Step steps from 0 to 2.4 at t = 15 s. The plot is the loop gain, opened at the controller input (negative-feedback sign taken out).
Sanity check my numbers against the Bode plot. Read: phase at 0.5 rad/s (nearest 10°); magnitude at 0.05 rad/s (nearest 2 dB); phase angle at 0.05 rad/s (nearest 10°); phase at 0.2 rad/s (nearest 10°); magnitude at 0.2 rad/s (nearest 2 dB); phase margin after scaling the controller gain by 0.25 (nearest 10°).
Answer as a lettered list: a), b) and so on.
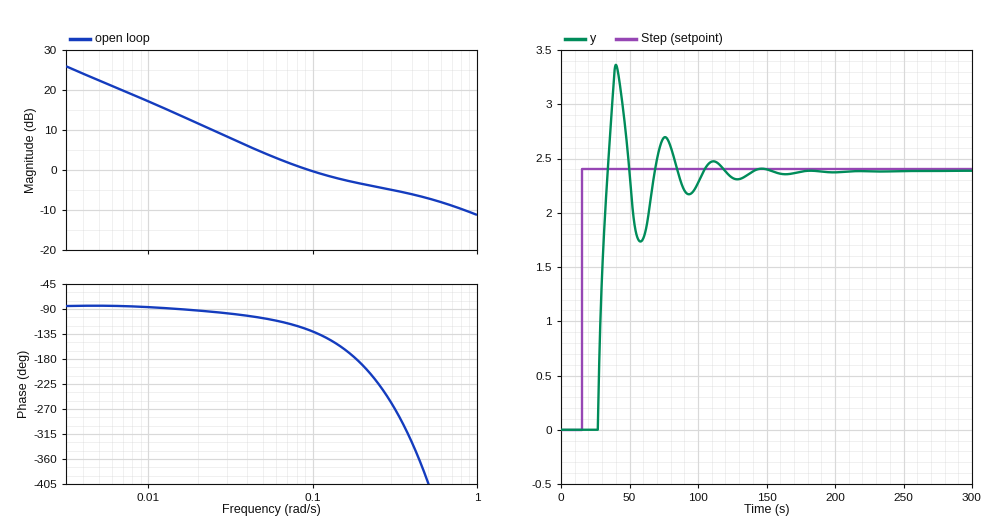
a) -400°
b) 4 dB
c) -110°
d) -190°
e) -4 dB
f) 90°
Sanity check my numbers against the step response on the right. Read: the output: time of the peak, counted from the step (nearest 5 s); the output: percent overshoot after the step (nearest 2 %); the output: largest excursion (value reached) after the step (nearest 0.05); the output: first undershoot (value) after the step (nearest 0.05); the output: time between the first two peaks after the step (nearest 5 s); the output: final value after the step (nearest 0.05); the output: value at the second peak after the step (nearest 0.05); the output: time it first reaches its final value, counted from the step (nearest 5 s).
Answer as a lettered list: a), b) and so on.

a) 25 s
b) 40 %
c) 3.35
d) 1.75
e) 35 s
f) 2.40
g) 2.70
h) 20 s
